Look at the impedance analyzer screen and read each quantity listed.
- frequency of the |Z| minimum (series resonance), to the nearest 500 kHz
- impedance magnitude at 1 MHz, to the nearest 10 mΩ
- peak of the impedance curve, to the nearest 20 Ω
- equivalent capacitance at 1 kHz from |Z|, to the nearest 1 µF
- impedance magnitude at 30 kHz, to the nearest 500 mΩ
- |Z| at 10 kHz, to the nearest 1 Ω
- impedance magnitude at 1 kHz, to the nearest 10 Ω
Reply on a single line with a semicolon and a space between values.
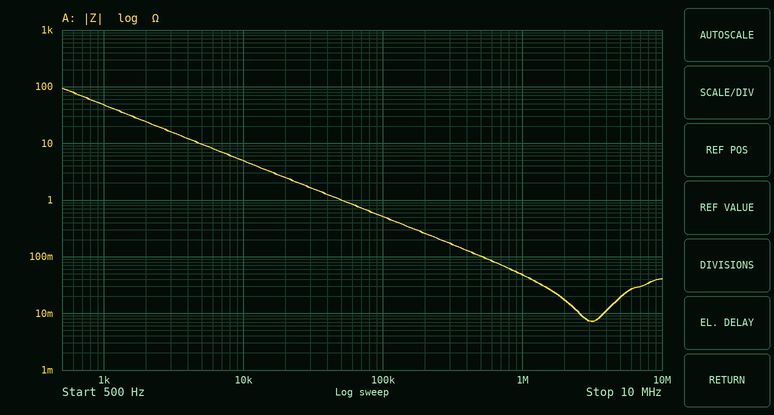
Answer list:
3.0 MHz; 50 mΩ; 100 Ω; 3 µF; 1.5 Ω; 5 Ω; 50 Ω
